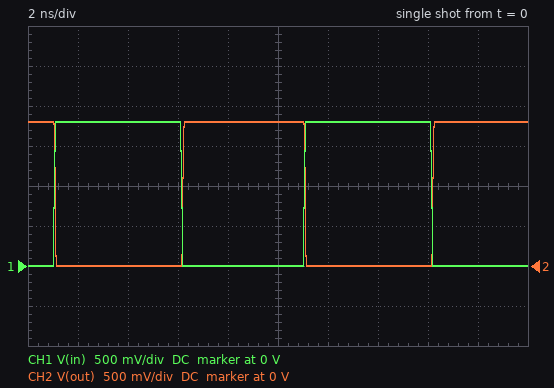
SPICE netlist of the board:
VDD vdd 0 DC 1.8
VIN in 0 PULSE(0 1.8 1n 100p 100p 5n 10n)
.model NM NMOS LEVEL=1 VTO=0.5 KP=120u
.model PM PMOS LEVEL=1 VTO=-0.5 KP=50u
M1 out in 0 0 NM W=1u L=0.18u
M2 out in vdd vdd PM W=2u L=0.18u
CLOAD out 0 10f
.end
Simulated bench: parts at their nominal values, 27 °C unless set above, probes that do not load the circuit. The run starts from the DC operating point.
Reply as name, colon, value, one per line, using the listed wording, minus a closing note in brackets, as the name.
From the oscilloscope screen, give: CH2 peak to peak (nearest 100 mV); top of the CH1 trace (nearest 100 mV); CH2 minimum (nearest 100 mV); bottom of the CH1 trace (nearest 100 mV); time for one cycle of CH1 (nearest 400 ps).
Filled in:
CH2 peak to peak: 1.8 V
top of the CH1 trace: 1.8 V
CH2 minimum: 0 V
bottom of the CH1 trace: 0 V
time for one cycle of CH1: 10.0 ns
